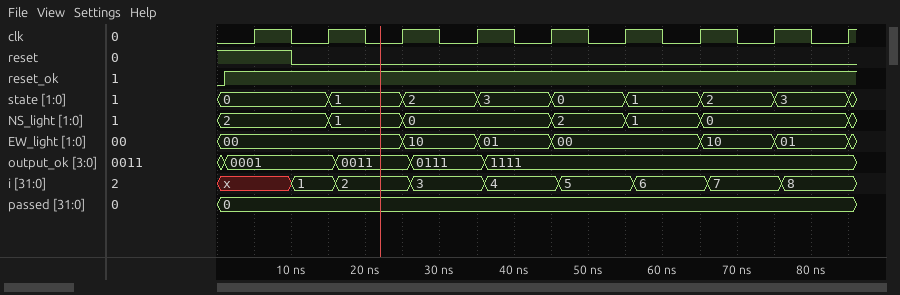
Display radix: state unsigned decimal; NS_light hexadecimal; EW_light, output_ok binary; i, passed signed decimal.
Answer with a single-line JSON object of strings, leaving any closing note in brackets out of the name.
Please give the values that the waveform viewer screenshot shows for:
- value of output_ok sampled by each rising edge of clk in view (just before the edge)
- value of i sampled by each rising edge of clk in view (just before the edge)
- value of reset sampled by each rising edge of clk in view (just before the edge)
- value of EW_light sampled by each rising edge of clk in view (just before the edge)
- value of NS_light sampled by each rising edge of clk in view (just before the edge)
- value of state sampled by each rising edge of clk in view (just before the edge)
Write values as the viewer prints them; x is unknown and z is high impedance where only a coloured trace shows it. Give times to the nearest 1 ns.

{"value of output_ok sampled by each rising edge of clk in view": "0001, 0001, 0011, 0111, 1111, 1111, 1111, 1111, 1111", "value of i sampled by each rising edge of clk in view": "x, 1, 2, 3, 4, 5, 6, 7, 8", "value of reset sampled by each rising edge of clk in view": "1 0 0 0 0 0 0 0 0", "value of EW_light sampled by each rising edge of clk in view": "00, 00, 00, 10, 01, 00, 00, 10, 01", "value of NS_light sampled by each rising edge of clk in view": "2, 2, 1, 0, 0, 2, 1, 0, 0", "value of state sampled by each rising edge of clk in view": "0, 0, 1, 2, 3, 0, 1, 2, 3"}
